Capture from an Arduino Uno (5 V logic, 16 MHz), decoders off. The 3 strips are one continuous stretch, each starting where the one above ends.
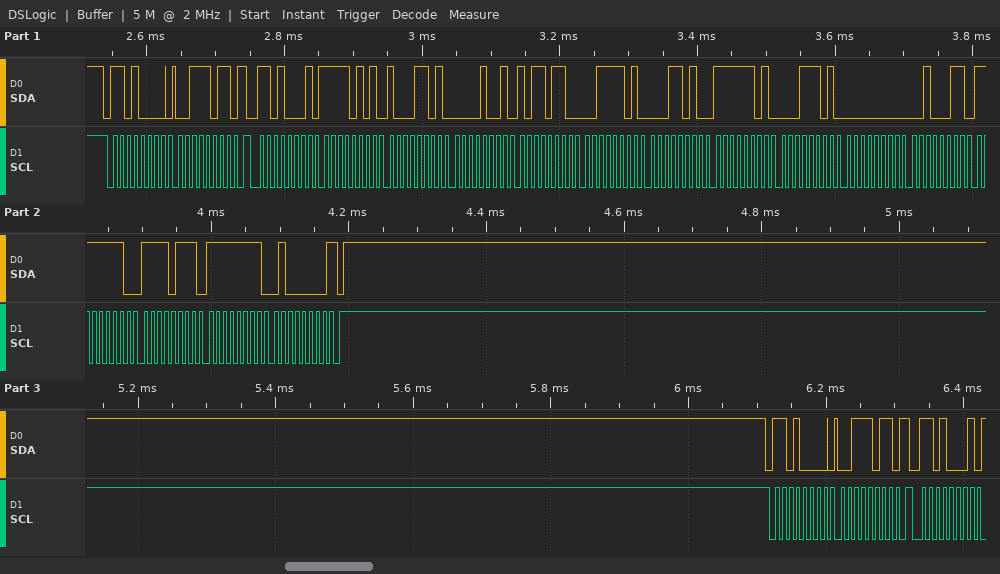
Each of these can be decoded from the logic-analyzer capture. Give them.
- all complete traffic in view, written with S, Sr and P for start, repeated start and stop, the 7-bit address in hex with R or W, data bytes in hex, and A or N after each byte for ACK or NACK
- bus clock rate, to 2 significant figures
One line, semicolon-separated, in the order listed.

S 68W A 3B A Sr 68R A F5 A 8D A 09 A B6 A 3D A 1A A FD A 1D A 00 A 23 A FE A F7 A FF A 40 N P S 68W A 3B A Sr 68R A; 100 kHz
